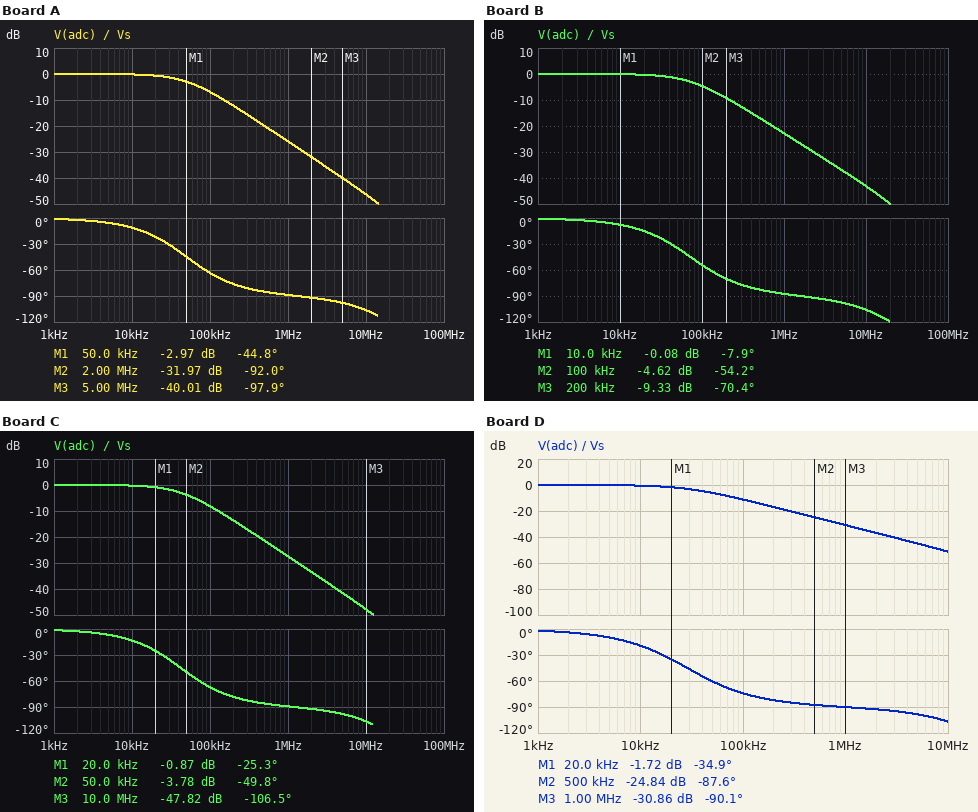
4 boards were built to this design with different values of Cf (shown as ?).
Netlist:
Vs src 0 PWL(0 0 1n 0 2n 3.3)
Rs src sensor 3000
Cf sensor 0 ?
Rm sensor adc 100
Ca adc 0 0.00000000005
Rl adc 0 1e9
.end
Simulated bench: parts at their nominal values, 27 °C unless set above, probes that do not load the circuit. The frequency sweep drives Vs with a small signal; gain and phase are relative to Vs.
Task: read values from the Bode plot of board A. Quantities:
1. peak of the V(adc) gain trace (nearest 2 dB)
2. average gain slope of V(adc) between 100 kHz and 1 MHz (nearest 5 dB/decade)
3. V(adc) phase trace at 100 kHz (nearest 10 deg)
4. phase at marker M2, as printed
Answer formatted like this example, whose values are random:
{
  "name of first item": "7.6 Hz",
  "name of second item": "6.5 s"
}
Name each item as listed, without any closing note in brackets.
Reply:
{
  "peak of the V(adc) gain trace": "0 dB",
  "average gain slope of V(adc) between 100 kHz and 1 MHz": "-20 dB/decade",
  "V(adc) phase trace at 100 kHz": "-60 deg",
  "phase at marker M2, as printed": "-92.0 deg"
}
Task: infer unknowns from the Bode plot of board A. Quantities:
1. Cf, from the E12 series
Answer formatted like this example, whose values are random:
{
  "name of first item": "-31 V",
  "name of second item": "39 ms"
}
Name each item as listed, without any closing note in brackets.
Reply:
{
  "Cf, from the E12 series": "1 nF"
}
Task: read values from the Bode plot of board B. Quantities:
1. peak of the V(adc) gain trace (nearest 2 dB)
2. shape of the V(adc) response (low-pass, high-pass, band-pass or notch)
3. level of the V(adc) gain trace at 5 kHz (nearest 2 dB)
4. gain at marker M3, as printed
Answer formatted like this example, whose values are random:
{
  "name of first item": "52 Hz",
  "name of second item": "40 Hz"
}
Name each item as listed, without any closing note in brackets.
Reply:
{
  "peak of the V(adc) gain trace": "0 dB",
  "shape of the V(adc) response": "low-pass",
  "level of the V(adc) gain trace at 5 kHz": "0 dB",
  "gain at marker M3, as printed": "-9.33 dB"
}
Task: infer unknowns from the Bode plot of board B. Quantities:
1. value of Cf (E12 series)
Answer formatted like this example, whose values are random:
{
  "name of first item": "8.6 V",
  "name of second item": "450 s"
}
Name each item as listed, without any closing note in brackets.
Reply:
{
  "value of Cf": "680 pF"
}
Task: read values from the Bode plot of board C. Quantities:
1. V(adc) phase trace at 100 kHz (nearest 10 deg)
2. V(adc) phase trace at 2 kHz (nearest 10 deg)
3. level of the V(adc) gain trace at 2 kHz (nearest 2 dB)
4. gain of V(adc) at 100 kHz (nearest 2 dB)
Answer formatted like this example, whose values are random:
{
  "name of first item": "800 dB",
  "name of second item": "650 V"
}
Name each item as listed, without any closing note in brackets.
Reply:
{
  "V(adc) phase trace at 100 kHz": "-70 deg",
  "V(adc) phase trace at 2 kHz": "0 deg",
  "level of the V(adc) gain trace at 2 kHz": "0 dB",
  "gain of V(adc) at 100 kHz": "-8 dB"
}
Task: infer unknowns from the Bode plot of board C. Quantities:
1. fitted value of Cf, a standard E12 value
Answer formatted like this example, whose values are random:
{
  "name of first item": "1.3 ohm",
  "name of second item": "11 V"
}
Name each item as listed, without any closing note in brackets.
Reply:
{
  "fitted value of Cf, a standard E12 value": "1.2 nF"
}
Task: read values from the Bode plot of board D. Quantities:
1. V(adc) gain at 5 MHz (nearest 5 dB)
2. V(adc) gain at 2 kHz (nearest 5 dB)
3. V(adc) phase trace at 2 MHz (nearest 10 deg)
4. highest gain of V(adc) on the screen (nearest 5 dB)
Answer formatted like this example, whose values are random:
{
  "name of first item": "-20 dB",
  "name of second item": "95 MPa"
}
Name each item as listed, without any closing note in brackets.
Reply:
{
  "V(adc) gain at 5 MHz": "-45 dB",
  "V(adc) gain at 2 kHz": "0 dB",
  "V(adc) phase trace at 2 MHz": "-90 deg",
  "highest gain of V(adc) on the screen": "0 dB"
}
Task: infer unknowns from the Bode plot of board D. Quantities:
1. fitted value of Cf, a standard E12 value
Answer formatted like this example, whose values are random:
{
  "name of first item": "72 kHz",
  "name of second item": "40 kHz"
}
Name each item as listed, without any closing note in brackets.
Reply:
{
  "fitted value of Cf, a standard E12 value": "1.8 nF"
}
